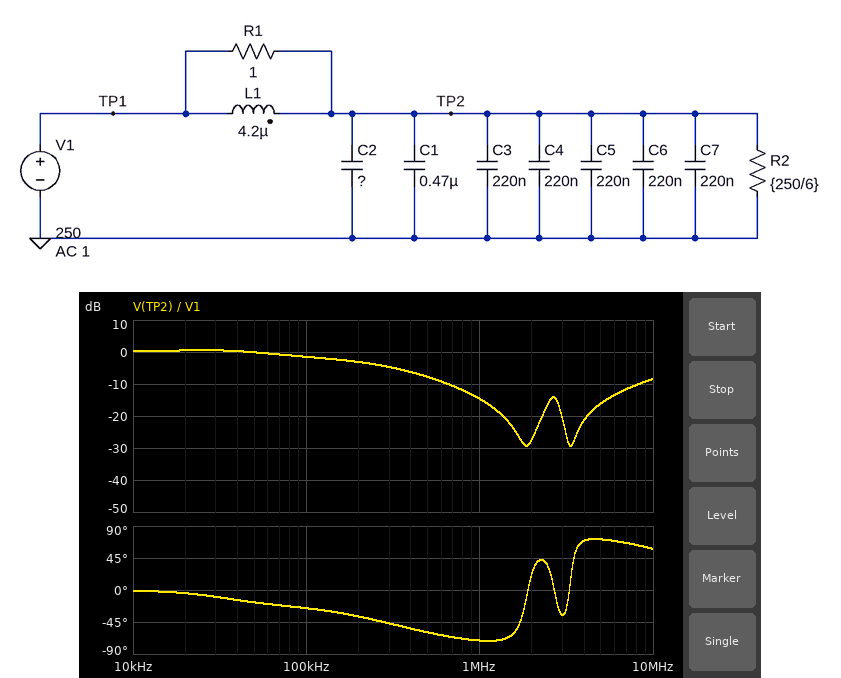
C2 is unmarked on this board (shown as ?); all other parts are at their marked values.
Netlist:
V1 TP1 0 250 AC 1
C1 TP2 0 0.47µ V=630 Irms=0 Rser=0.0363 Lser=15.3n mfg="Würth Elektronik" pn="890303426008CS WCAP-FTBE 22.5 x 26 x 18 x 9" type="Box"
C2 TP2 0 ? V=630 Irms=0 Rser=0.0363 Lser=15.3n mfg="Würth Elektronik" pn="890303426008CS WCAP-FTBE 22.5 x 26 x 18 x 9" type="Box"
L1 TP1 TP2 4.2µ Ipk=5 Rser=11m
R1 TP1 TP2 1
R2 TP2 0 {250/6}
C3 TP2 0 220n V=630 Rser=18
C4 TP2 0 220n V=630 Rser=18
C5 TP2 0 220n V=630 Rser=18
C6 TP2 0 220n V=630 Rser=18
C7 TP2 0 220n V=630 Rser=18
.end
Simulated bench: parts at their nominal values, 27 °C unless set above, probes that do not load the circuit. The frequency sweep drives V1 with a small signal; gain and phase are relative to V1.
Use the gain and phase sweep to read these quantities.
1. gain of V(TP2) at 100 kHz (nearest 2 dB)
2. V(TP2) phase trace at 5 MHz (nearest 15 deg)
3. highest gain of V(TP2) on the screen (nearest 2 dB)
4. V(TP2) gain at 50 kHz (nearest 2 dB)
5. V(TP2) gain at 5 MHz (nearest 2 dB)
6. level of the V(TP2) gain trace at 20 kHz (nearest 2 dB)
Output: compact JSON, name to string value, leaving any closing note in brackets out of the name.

{"gain of V(TP2) at 100 kHz": "-2 dB", "V(TP2) phase trace at 5 MHz": "75 deg", "highest gain of V(TP2) on the screen": "0 dB", "V(TP2) gain at 50 kHz": "0 dB", "V(TP2) gain at 5 MHz": "-16 dB", "level of the V(TP2) gain trace at 20 kHz": "0 dB"}
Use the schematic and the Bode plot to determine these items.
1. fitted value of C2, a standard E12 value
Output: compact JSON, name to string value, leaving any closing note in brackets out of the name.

{"fitted value of C2, a standard E12 value": "150 nF"}
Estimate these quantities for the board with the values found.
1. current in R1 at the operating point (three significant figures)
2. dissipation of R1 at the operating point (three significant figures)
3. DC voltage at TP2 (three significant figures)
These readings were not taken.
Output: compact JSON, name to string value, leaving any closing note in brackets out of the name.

{"current in R1 at the operating point": "65.3 mA", "dissipation of R1 at the operating point": "4.26 mW", "DC voltage at TP2": "250 V"}
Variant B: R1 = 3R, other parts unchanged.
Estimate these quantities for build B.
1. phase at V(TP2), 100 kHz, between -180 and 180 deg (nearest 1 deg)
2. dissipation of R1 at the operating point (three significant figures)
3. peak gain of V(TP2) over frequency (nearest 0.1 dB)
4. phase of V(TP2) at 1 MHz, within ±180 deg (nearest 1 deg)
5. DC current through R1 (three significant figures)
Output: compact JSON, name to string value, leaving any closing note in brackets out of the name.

{"phase at V(TP2), 100 kHz, between -180 and 180 deg": "-59 deg", "dissipation of R1 at the operating point": "1.44 mW", "peak gain of V(TP2) over frequency": "1.8 dB", "phase of V(TP2) at 1 MHz, within ±180 deg": "-82 deg", "DC current through R1": "21.9 mA"}
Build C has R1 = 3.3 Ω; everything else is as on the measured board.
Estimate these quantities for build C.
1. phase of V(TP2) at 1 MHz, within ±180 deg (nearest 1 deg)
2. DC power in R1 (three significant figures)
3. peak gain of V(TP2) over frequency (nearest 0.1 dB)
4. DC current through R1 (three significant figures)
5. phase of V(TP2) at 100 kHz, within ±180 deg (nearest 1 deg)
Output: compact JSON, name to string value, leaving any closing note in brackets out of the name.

{"phase of V(TP2) at 1 MHz, within ±180 deg": "-83 deg", "DC power in R1": "1.31 mW", "peak gain of V(TP2) over frequency": "1.9 dB", "DC current through R1": "19.9 mA", "phase of V(TP2) at 100 kHz, within ±180 deg": "-62 deg"}
